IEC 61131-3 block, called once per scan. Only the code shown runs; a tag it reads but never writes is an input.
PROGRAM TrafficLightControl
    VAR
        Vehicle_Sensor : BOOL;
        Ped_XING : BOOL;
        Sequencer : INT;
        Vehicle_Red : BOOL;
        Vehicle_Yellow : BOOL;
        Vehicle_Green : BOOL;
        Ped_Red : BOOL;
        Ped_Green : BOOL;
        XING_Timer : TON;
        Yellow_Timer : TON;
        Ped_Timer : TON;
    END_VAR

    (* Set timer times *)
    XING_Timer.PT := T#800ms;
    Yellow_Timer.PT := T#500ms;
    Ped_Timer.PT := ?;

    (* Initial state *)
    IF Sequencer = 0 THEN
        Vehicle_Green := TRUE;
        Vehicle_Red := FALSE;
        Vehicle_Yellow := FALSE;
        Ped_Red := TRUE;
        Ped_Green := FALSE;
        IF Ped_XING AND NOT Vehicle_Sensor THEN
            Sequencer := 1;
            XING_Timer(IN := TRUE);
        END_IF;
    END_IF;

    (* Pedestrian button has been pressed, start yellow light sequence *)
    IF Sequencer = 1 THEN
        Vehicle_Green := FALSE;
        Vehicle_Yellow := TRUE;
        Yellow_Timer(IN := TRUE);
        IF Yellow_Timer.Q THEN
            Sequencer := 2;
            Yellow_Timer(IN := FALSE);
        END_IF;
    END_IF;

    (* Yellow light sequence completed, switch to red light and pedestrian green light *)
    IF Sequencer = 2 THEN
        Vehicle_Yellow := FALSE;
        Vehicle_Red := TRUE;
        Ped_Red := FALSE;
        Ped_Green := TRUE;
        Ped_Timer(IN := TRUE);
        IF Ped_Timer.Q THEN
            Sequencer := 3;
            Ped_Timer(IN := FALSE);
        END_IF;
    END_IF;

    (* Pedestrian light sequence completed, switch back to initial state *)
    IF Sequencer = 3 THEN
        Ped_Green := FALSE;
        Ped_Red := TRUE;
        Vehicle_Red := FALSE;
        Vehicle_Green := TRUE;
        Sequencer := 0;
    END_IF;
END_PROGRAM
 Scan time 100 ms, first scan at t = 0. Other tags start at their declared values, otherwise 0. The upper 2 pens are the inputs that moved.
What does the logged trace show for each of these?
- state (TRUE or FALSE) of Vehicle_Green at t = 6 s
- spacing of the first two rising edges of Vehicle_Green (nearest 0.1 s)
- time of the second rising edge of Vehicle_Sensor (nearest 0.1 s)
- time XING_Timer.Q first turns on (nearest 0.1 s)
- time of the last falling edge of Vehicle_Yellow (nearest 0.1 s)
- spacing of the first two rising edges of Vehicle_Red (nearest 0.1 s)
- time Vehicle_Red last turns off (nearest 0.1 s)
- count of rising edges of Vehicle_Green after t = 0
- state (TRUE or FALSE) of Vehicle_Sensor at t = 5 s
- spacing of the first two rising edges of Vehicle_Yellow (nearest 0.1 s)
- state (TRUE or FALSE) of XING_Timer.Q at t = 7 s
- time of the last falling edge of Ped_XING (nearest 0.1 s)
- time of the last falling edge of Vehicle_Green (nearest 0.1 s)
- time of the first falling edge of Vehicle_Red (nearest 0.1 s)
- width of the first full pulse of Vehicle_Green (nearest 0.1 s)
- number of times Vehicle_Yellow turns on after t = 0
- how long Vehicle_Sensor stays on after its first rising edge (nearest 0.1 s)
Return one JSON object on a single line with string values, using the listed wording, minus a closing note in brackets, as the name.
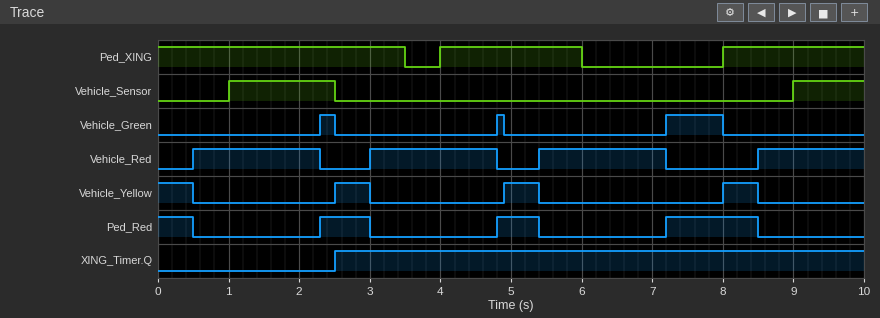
{"state (TRUE or FALSE) of Vehicle_Green at t = 6 s": "FALSE", "spacing of the first two rising edges of Vehicle_Green": "2.5 s", "time of the second rising edge of Vehicle_Sensor": "9.0 s", "time XING_Timer.Q first turns on": "2.5 s", "time of the last falling edge of Vehicle_Yellow": "8.5 s", "spacing of the first two rising edges of Vehicle_Red": "2.5 s", "time Vehicle_Red last turns off": "7.2 s", "count of rising edges of Vehicle_Green after t = 0": "3", "state (TRUE or FALSE) of Vehicle_Sensor at t = 5 s": "FALSE", "spacing of the first two rising edges of Vehicle_Yellow": "2.4 s", "state (TRUE or FALSE) of XING_Timer.Q at t = 7 s": "TRUE", "time of the last falling edge of Ped_XING": "6.0 s", "time of the last falling edge of Vehicle_Green": "8.0 s", "time of the first falling edge of Vehicle_Red": "2.3 s", "width of the first full pulse of Vehicle_Green": "0.2 s", "number of times Vehicle_Yellow turns on after t = 0": "3", "how long Vehicle_Sensor stays on after its first rising edge": "1.5 s"}
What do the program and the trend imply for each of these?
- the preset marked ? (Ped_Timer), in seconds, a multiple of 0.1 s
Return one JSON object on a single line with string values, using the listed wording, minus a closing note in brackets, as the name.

{"the preset marked ? (Ped_Timer), in seconds, a multiple of 0.1 s": "1.8 s"}
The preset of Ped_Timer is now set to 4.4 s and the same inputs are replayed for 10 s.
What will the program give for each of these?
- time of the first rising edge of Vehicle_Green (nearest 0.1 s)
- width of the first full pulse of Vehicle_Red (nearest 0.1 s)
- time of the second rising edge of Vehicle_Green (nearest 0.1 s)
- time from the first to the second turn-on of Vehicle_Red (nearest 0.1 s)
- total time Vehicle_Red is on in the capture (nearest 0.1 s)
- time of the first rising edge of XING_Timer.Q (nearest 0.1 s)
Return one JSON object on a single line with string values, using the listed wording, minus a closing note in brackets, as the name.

{"time of the first rising edge of Vehicle_Green": "4.9 s", "width of the first full pulse of Vehicle_Red": "4.4 s", "time of the second rising edge of Vehicle_Green": "9.9 s", "time from the first to the second turn-on of Vehicle_Red": "5.0 s", "total time Vehicle_Red is on in the capture": "8.8 s", "time of the first rising edge of XING_Timer.Q": "5.0 s"}
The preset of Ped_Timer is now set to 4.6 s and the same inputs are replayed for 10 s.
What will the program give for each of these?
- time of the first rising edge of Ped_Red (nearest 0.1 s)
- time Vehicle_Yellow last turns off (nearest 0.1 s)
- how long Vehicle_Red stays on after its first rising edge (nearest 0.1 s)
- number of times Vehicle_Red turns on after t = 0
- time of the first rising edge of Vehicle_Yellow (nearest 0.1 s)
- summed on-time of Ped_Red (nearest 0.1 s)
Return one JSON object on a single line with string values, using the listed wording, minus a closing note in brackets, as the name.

{"time of the first rising edge of Ped_Red": "5.1 s", "time Vehicle_Yellow last turns off": "5.7 s", "how long Vehicle_Red stays on after its first rising edge": "4.6 s", "number of times Vehicle_Red turns on after t = 0": "2", "time of the first rising edge of Vehicle_Yellow": "5.2 s", "summed on-time of Ped_Red": "1.1 s"}
